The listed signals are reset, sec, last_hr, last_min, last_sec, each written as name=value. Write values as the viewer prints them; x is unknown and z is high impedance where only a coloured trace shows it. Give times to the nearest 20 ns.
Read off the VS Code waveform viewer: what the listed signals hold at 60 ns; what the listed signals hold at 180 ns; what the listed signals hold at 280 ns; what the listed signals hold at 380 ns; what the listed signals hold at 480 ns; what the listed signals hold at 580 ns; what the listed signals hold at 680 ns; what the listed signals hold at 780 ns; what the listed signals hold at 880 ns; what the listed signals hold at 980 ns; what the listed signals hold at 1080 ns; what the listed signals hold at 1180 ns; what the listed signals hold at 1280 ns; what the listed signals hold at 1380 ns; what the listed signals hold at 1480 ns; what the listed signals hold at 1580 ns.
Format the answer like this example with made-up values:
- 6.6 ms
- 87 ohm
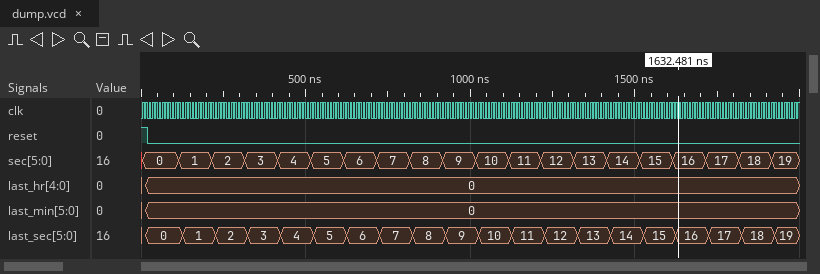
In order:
- reset=0, sec=0, last_hr=0, last_min=0, last_sec=0
- reset=0, sec=1, last_hr=0, last_min=0, last_sec=1
- reset=0, sec=2, last_hr=0, last_min=0, last_sec=2
- reset=0, sec=3, last_hr=0, last_min=0, last_sec=3
- reset=0, sec=4, last_hr=0, last_min=0, last_sec=4
- reset=0, sec=5, last_hr=0, last_min=0, last_sec=5
- reset=0, sec=6, last_hr=0, last_min=0, last_sec=6
- reset=0, sec=7, last_hr=0, last_min=0, last_sec=7
- reset=0, sec=8, last_hr=0, last_min=0, last_sec=8
- reset=0, sec=9, last_hr=0, last_min=0, last_sec=9
- reset=0, sec=10, last_hr=0, last_min=0, last_sec=10
- reset=0, sec=11, last_hr=0, last_min=0, last_sec=11
- reset=0, sec=12, last_hr=0, last_min=0, last_sec=12
- reset=0, sec=13, last_hr=0, last_min=0, last_sec=13
- reset=0, sec=14, last_hr=0, last_min=0, last_sec=14
- reset=0, sec=15, last_hr=0, last_min=0, last_sec=15
